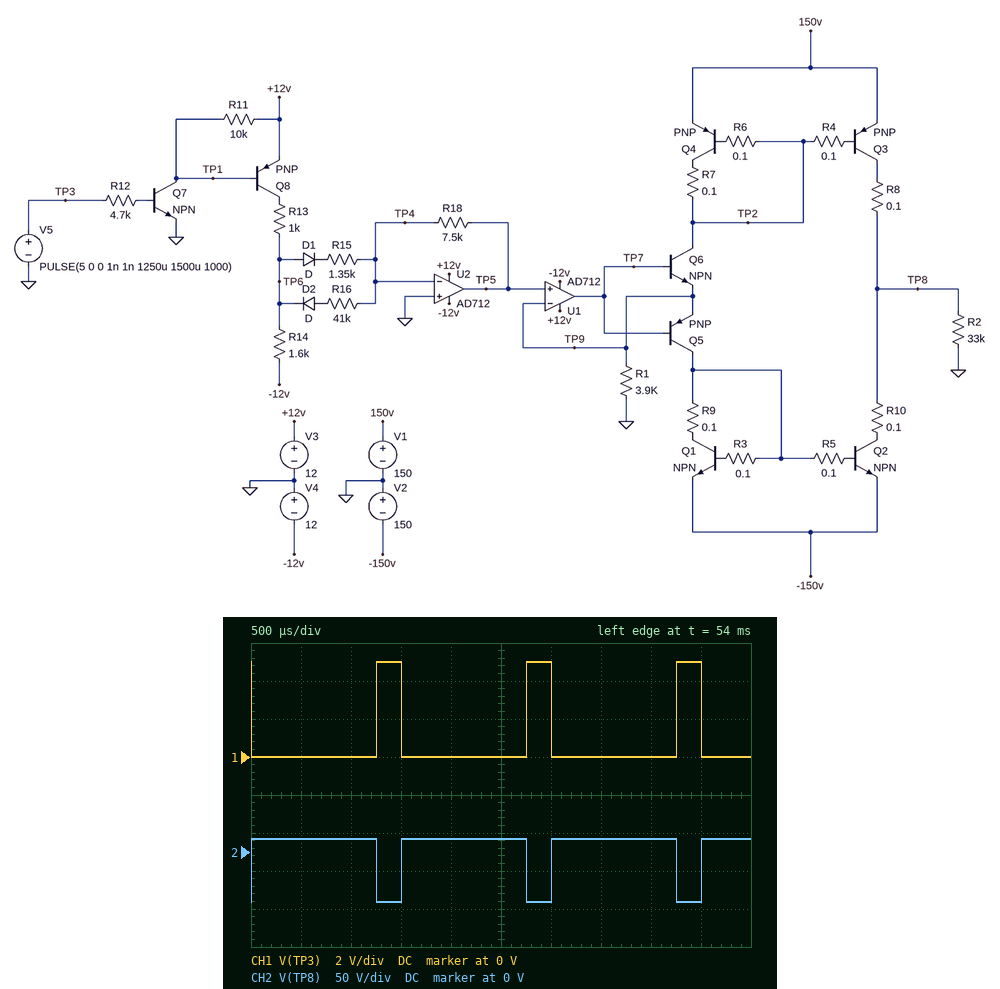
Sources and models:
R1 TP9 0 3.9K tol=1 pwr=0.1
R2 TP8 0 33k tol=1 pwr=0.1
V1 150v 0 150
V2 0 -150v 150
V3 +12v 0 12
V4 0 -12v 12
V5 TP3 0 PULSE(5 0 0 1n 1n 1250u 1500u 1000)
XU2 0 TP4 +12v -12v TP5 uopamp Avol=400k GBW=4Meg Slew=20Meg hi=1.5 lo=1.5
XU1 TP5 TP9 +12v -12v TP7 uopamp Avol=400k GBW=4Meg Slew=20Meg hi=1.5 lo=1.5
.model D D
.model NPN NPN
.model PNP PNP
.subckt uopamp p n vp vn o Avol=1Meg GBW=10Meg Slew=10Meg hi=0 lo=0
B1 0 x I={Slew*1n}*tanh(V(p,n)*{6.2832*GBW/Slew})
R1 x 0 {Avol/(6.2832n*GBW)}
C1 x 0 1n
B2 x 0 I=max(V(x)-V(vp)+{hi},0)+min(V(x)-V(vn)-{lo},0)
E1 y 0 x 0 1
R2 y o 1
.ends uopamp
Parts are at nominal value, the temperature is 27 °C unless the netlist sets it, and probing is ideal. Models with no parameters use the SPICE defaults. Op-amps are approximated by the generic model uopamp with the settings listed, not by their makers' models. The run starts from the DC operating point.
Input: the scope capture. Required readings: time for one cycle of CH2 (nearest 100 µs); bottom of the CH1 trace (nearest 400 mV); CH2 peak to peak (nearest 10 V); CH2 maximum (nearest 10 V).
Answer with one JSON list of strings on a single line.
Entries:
["1.5 ms", "0 V", "80 V", "20 V"]
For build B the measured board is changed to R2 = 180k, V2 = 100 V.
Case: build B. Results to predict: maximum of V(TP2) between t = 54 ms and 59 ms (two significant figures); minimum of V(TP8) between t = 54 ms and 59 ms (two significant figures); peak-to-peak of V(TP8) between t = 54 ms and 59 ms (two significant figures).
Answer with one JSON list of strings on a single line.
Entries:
["150 V", "-100 V", "190 V"]
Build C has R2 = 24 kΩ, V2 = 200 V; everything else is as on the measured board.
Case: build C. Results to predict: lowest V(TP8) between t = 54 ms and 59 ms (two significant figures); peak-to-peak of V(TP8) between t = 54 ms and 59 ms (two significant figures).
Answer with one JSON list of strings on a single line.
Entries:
["-48 V", "60 V"]
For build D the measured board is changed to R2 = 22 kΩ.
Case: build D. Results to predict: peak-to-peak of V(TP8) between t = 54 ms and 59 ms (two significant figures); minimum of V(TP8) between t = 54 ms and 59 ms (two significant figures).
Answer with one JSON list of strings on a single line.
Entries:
["55 V", "-44 V"]
